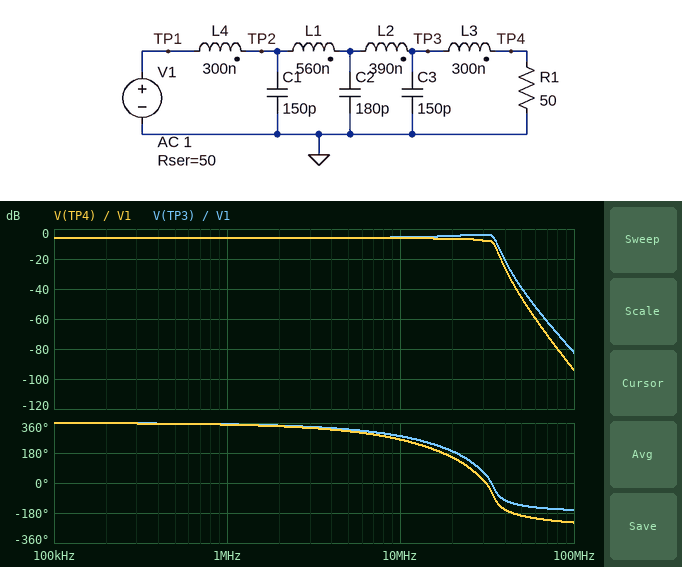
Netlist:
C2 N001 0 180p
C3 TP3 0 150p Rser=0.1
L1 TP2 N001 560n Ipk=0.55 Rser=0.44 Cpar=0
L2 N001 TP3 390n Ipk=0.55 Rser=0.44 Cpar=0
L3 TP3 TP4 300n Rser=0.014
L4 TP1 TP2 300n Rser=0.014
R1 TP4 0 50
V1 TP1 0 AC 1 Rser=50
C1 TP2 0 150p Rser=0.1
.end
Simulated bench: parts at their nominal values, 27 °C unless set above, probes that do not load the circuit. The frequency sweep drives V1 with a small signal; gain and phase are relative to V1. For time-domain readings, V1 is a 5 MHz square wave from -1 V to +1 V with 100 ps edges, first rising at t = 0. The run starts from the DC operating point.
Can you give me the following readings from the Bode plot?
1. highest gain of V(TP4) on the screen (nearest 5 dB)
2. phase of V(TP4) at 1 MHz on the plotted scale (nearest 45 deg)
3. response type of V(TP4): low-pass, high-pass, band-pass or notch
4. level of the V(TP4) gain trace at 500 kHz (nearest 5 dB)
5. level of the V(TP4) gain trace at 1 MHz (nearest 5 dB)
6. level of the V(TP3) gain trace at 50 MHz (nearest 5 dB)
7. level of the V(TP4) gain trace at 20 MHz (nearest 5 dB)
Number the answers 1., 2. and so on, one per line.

1. -5 dB
2. 360 deg
3. low-pass
4. -5 dB
5. -5 dB
6. -40 dB
7. -5 dB
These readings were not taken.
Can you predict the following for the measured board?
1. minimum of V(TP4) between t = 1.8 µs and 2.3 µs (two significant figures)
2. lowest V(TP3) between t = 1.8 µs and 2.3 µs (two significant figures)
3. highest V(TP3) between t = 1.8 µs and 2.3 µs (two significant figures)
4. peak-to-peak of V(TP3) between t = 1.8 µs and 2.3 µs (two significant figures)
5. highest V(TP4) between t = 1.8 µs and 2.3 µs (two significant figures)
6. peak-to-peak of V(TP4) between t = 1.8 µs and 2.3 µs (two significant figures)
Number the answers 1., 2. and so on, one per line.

1. -660 mV
2. -790 mV
3. 790 mV
4. 1.6 V
5. 660 mV
6. 1.3 V
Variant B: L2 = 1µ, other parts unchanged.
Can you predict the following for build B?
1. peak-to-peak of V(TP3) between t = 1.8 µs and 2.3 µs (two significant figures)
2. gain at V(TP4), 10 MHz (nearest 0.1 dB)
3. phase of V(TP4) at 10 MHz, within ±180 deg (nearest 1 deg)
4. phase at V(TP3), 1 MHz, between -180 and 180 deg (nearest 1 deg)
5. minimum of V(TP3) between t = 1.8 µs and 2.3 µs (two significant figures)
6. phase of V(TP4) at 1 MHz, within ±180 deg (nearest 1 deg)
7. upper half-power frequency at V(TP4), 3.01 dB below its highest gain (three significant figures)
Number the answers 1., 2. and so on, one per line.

1. 1.4 V
2. -6.5 dB
3. -118 deg
4. -10 deg
5. -690 mV
6. -12 deg
7. 24.8 MHz
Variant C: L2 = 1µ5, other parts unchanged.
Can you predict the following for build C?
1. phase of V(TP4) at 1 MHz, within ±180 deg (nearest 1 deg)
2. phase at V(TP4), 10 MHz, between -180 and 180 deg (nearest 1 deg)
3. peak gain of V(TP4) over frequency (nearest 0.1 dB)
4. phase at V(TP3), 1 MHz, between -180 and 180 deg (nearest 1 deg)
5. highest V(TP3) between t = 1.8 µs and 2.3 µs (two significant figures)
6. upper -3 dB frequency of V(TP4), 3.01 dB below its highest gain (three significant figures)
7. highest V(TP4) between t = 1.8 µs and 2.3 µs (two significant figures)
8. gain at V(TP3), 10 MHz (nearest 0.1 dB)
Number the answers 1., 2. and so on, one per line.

1. -14 deg
2. -131 deg
3. -6.1 dB
4. -12 deg
5. 570 mV
6. 17.2 MHz
7. 520 mV
8. -6.7 dB
